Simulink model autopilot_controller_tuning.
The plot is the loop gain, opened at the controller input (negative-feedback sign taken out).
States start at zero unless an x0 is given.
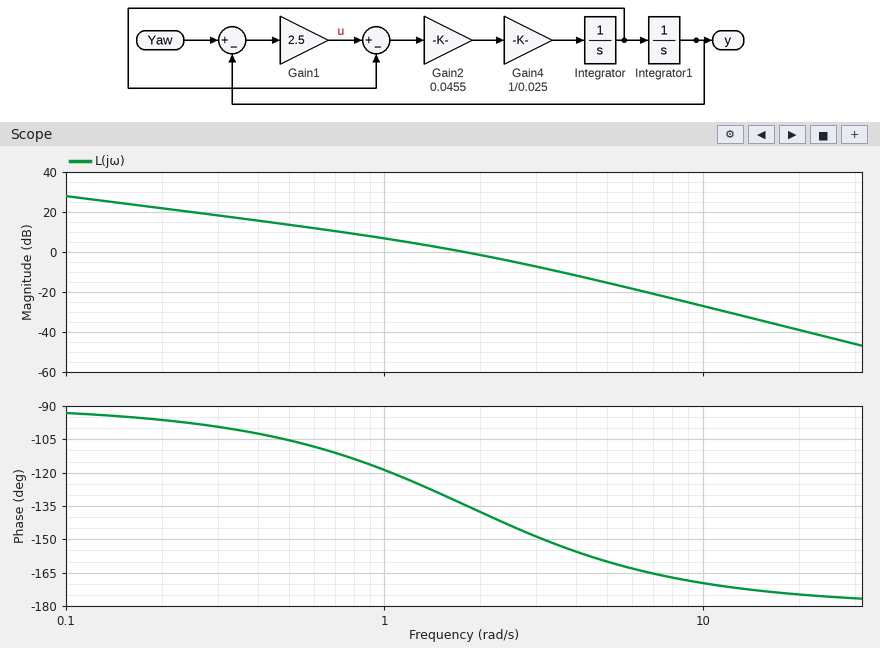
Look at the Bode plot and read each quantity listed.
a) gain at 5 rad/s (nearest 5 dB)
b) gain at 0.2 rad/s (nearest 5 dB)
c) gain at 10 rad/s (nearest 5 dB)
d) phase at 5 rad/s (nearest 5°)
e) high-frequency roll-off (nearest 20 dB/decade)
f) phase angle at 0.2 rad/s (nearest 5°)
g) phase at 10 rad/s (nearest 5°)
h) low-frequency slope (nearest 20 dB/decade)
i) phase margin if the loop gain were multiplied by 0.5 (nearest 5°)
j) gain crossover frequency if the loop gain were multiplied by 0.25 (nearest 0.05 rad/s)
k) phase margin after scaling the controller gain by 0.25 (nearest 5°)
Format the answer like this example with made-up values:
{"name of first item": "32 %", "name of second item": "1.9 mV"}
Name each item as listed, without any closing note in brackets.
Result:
{"gain at 5 rad/s": "-15 dB", "gain at 0.2 rad/s": "20 dB", "gain at 10 rad/s": "-25 dB", "phase at 5 rad/s": "-160°", "high-frequency roll-off": "-40 dB/decade", "phase angle at 0.2 rad/s": "-95°", "phase at 10 rad/s": "-170°", "low-frequency slope": "-20 dB/decade", "phase margin if the loop gain were multiplied by 0.5": "60°", "gain crossover frequency if the loop gain were multiplied by 0.25": "0.60 rad/s", "phase margin after scaling the controller gain by 0.25": "70°"}
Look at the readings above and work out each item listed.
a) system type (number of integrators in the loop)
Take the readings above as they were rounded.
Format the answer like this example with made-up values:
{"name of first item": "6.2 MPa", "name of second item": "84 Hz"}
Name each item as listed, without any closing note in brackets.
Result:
{"system type": "1"}
